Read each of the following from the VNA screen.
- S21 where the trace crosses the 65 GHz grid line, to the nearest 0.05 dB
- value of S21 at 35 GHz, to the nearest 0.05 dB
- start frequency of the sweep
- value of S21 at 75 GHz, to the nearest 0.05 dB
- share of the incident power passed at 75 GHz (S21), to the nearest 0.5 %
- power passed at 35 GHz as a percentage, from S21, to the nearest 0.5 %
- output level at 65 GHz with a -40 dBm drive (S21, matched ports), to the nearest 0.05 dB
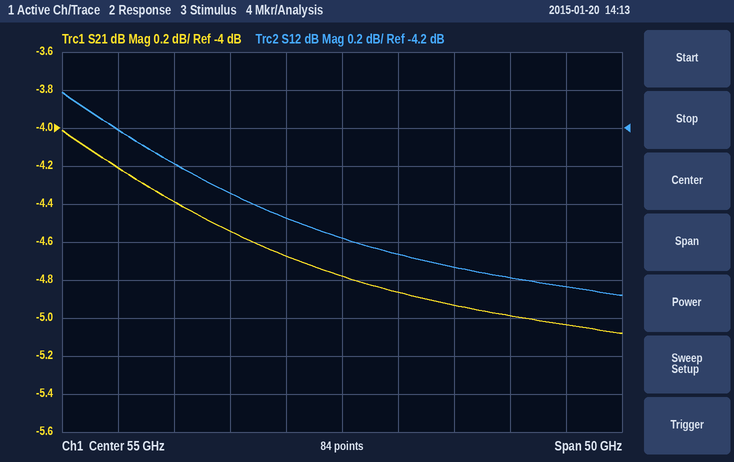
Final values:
-4.95 dB
-4.20 dB
30 GHz
-5.05 dB
31.5 %
38.0 %
-44.95 dBm
